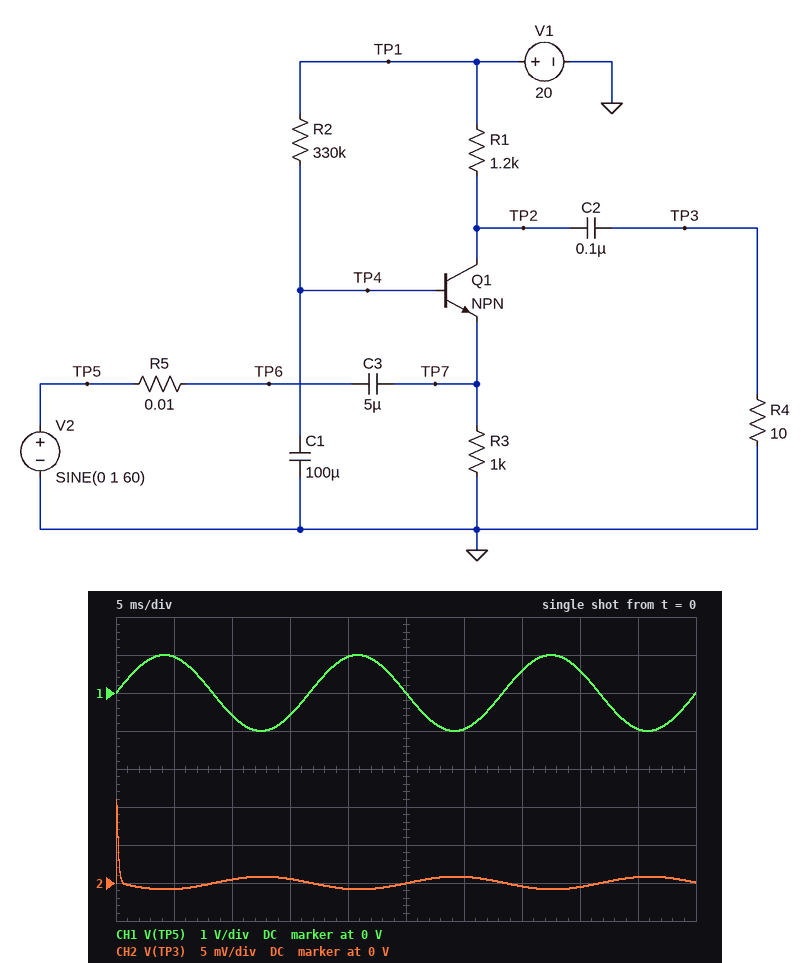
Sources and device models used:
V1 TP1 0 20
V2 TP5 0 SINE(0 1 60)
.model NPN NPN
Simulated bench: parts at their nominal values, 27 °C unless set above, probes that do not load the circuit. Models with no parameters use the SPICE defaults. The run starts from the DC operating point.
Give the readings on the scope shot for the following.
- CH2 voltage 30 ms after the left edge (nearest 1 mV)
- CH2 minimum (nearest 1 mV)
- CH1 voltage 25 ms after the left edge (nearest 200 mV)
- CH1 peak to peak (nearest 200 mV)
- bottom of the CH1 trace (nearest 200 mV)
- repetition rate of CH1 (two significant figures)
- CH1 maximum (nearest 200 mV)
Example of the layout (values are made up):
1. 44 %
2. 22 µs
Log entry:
1. 1 mV
2. -1 mV
3. 0 V
4. 2.0 V
5. -1.0 V
6. 60 Hz
7. 1.0 V
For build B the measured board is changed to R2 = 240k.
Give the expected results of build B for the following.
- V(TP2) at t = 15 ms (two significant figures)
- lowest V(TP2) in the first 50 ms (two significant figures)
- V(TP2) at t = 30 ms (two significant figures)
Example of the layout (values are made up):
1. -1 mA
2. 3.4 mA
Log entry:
1. 15 V
2. 11 V
3. 14 V
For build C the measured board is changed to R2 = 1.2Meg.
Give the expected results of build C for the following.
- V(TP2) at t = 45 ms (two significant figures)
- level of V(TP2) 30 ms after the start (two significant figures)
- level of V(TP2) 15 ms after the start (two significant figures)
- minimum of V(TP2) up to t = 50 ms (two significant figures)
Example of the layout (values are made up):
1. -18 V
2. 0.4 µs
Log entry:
1. 17 V
2. 19 V
3. 20 V
4. 16 V
